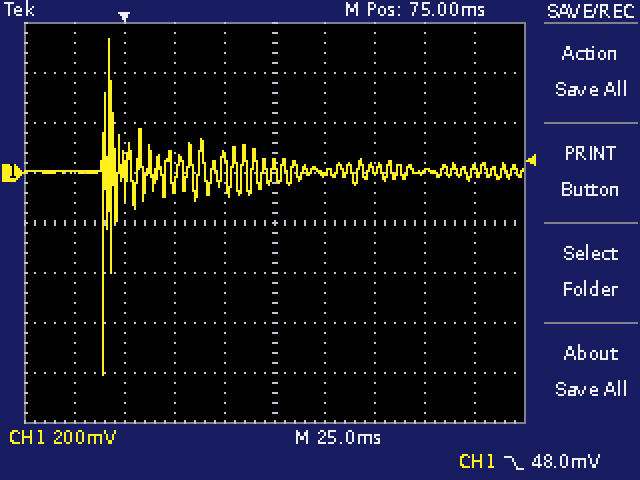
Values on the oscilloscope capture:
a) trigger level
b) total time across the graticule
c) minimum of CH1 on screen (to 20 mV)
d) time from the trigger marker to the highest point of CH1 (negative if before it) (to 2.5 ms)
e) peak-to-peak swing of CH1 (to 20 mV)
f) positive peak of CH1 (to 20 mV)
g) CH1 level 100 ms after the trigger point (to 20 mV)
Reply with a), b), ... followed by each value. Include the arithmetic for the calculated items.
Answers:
a) 48.0 mV
b) 250 ms
c) -800 mV
d) -7.5 ms
e) 540 mV − (-800 mV) = 1.34 V
f) 540 mV
g) 0 mV
